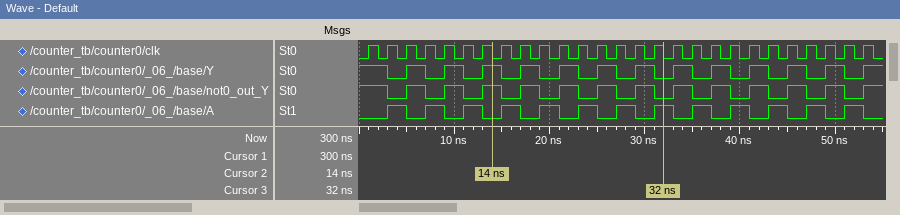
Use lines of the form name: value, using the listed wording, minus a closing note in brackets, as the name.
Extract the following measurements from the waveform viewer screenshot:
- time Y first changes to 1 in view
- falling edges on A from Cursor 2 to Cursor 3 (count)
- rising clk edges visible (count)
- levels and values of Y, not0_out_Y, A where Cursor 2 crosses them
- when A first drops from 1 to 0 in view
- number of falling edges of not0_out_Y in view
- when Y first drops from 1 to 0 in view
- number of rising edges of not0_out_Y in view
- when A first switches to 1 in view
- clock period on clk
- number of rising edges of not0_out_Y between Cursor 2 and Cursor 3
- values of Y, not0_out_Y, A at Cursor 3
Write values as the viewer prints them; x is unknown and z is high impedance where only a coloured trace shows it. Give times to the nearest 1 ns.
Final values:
time Y first changes to 1 in view: 5 ns
falling edges on A from Cursor 2 to Cursor 3: 4
rising clk edges visible: 27
levels and values of Y, not0_out_Y, A where Cursor 2 crosses them: Y=1, not0_out_Y=1, A=0
when A first drops from 1 to 0 in view: 5 ns
number of falling edges of not0_out_Y in view: 13
when Y first drops from 1 to 0 in view: 3 ns
number of rising edges of not0_out_Y in view: 13
when A first switches to 1 in view: 3 ns
clock period on clk: 2 ns
number of rising edges of not0_out_Y between Cursor 2 and Cursor 3: 4
values of Y, not0_out_Y, A at Cursor 3: Y=0, not0_out_Y=0, A=1
